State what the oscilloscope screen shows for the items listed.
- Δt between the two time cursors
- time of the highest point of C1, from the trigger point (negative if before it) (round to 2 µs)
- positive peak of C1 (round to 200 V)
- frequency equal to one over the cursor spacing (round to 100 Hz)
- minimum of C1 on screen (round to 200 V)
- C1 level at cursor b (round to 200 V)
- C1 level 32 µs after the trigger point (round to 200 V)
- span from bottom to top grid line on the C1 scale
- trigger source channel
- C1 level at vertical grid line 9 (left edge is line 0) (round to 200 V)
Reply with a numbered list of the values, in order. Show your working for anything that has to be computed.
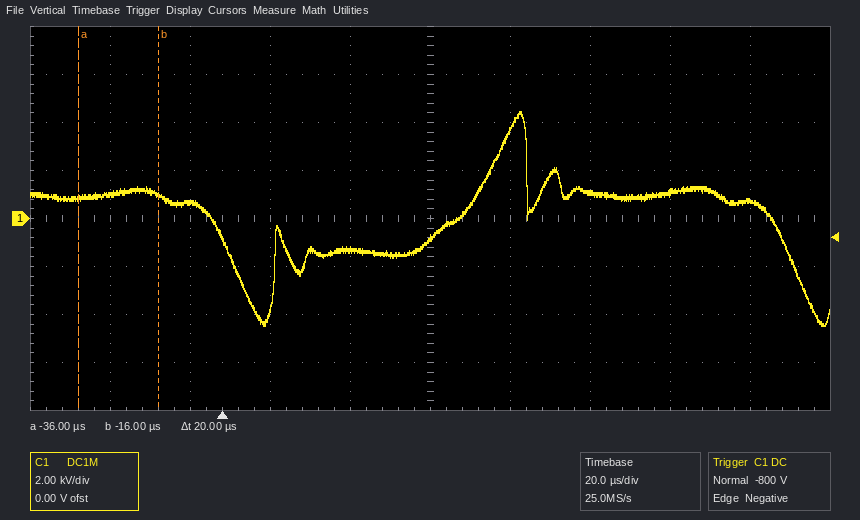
1. 20 µs
2. +74 µs
3. 4.4 kV
4. 1 / 20 µs ≈ 50.0 kHz
5. -4.4 kV
6. 1.0 kV
7. -1.2 kV
8. 16 kV
9. C1
10. 800 V
